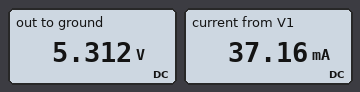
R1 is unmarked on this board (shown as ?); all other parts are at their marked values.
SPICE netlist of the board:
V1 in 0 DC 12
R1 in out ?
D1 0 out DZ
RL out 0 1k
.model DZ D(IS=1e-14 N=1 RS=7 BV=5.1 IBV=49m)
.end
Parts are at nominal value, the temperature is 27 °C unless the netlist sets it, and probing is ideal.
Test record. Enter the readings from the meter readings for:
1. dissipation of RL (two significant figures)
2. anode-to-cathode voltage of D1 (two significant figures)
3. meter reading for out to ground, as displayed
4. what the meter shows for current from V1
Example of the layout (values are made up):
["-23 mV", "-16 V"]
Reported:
["28 mW", "-5.3 V", "5.312 V", "37.16 mA"]
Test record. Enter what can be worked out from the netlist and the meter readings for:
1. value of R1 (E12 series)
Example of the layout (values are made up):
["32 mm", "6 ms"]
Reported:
["180 Ω"]
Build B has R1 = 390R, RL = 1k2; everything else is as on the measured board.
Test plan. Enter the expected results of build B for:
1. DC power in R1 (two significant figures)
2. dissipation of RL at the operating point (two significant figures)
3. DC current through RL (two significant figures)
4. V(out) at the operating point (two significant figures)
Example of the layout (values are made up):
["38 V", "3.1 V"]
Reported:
["120 mW", "22 mW", "4.3 mA", "5.2 V"]
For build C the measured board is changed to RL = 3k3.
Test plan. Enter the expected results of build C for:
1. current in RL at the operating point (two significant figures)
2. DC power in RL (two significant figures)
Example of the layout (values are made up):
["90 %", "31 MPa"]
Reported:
["1.6 mA", "8.6 mW"]
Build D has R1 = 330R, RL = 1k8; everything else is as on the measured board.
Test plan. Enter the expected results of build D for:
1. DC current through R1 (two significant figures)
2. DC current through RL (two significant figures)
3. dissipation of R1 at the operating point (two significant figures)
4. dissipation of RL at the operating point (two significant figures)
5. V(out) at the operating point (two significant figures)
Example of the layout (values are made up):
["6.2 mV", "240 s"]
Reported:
["21 mA", "2.9 mA", "140 mW", "15 mW", "5.2 V"]
